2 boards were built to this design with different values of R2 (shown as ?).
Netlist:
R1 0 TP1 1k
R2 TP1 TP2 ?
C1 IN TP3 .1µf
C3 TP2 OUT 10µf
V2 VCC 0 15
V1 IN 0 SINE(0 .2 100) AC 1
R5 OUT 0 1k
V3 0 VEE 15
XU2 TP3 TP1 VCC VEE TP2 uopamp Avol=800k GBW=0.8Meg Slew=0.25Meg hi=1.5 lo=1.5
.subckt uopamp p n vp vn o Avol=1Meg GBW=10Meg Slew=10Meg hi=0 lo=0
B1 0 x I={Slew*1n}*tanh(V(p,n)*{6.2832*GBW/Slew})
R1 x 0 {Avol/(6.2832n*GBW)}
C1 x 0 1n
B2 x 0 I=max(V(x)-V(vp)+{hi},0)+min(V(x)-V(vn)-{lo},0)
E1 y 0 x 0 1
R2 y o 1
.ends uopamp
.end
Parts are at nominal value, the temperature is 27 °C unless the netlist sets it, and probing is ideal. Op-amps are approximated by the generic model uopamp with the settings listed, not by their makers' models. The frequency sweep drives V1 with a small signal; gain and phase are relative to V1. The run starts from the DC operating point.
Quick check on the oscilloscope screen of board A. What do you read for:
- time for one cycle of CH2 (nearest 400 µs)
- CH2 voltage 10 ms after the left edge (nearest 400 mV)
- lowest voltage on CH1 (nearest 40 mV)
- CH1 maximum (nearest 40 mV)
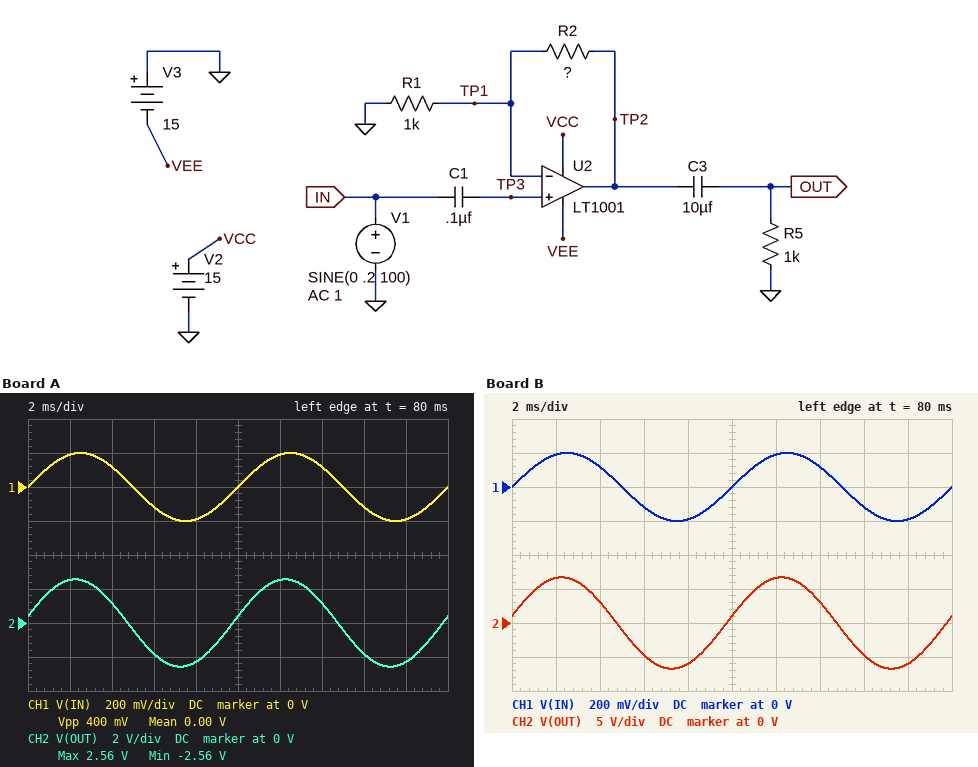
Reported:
10.0 ms
400 mV
-200 mV
200 mV
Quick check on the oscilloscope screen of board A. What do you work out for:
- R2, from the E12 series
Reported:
12 kΩ
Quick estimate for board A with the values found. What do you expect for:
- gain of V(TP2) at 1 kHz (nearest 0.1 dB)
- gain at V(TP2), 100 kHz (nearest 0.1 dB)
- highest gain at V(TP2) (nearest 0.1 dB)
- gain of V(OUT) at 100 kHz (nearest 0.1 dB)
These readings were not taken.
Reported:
22.3 dB
16.7 dB
22.3 dB
16.7 dB
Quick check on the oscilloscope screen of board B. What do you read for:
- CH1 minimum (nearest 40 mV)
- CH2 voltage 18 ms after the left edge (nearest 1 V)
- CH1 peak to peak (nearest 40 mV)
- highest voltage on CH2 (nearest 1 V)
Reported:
-200 mV
-6 V
400 mV
7 V
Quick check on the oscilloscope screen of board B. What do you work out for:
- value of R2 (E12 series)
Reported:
33 kΩ
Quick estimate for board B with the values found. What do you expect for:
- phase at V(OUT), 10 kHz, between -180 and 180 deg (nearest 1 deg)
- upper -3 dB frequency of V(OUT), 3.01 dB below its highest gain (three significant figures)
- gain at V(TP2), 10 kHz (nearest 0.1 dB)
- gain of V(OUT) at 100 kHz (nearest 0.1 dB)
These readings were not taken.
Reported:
-23 deg
23.5 kHz
29.9 dB
17.8 dB
